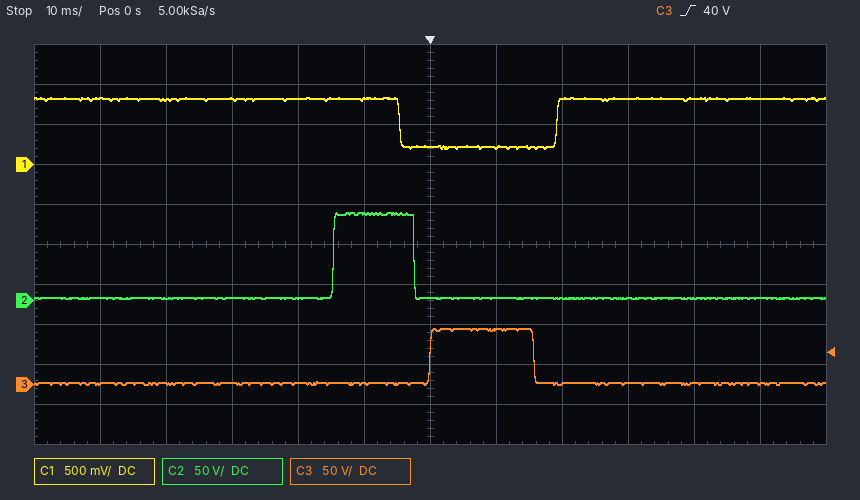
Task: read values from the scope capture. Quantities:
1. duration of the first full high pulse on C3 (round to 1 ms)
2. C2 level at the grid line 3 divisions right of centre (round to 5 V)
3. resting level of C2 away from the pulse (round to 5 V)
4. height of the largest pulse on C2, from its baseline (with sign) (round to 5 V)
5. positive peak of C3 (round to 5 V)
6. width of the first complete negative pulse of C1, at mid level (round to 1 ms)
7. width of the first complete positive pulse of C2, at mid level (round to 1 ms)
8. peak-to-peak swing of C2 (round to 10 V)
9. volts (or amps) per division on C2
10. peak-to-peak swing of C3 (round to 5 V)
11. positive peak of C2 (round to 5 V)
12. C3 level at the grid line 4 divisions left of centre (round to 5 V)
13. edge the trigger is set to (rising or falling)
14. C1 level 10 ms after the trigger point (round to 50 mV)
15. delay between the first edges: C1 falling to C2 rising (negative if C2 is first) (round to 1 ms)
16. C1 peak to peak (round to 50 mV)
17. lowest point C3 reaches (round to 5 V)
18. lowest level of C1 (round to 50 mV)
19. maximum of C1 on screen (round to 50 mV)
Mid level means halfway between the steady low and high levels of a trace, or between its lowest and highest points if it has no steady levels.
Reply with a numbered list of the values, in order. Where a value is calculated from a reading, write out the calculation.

1. 16 ms
2. 5 V
3. 5 V
4. 110 V − (5 V) = +105 V
5. 70 V
6. 24 ms
7. 12 ms
8. 110 V
9. 50 V
10. 70 V − (0 V) = 70 V
11. 110 V
12. 0 V
13. rising
14. 200 mV
15. -10 ms
16. 850 mV − (200 mV) = 650 mV
17. 0 V
18. 200 mV
19. 850 mV
